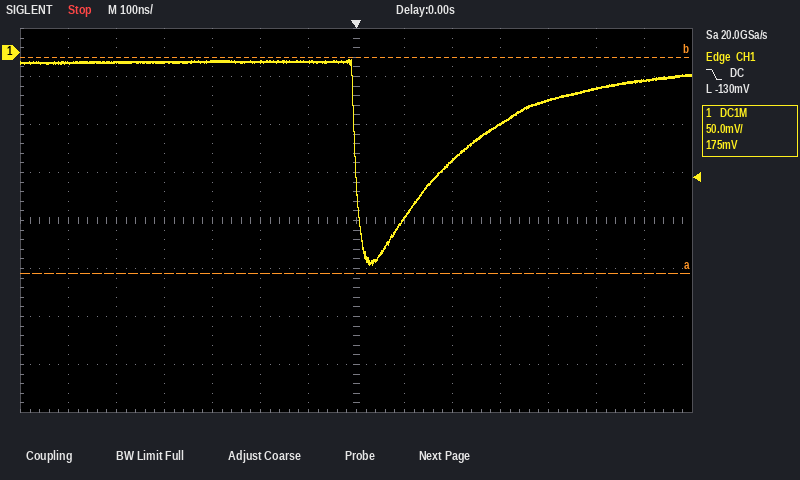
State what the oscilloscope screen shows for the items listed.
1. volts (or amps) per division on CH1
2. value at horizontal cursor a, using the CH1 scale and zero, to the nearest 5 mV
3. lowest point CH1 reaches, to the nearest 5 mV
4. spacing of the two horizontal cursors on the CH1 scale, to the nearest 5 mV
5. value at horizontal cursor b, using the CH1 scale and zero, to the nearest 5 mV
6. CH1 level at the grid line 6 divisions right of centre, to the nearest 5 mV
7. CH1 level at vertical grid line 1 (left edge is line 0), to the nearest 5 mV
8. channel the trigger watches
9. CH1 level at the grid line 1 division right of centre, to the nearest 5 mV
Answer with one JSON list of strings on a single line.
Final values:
["50 mV", "-230 mV", "-220 mV", "225 mV", "-5 mV", "-30 mV", "-10 mV", "CH1", "-175 mV"]
